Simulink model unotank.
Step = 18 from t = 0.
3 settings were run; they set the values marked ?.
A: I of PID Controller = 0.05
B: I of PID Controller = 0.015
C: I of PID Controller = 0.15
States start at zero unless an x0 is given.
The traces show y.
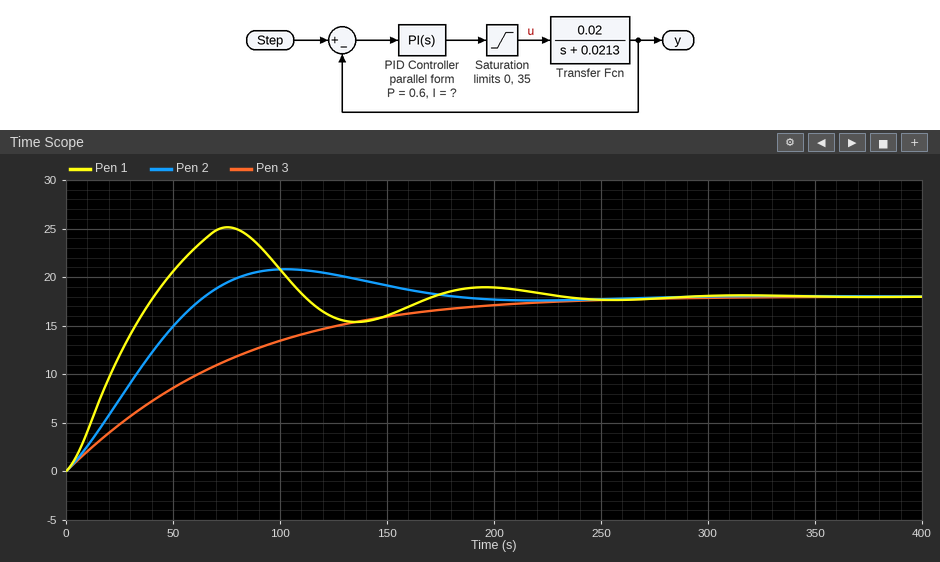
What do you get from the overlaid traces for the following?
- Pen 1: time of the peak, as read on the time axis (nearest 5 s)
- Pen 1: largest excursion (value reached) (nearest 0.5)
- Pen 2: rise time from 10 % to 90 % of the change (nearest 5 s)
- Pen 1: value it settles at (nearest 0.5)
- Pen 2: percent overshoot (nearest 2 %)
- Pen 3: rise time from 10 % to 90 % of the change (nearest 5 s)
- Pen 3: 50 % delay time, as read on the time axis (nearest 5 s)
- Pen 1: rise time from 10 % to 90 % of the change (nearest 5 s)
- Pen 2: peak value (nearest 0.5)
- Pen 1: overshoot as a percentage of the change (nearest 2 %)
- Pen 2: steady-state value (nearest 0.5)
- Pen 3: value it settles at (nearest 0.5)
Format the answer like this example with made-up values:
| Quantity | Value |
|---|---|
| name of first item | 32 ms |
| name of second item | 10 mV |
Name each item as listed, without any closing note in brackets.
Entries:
| Quantity | Value |
|---|---|
| Pen 1: time of the peak, as read on the time axis | 75 s |
| Pen 1: largest excursion (value reached) | 25.0 |
| Pen 2: rise time from 10 % to 90 % of the change | 50 s |
| Pen 1: value it settles at | 18.0 |
| Pen 2: percent overshoot | 16 % |
| Pen 3: rise time from 10 % to 90 % of the change | 150 s |
| Pen 3: 50 % delay time, as read on the time axis | 55 s |
| Pen 1: rise time from 10 % to 90 % of the change | 30 s |
| Pen 2: peak value | 21.0 |
| Pen 1: overshoot as a percentage of the change | 40 % |
| Pen 2: steady-state value | 18.0 |
| Pen 3: value it settles at | 18.0 |
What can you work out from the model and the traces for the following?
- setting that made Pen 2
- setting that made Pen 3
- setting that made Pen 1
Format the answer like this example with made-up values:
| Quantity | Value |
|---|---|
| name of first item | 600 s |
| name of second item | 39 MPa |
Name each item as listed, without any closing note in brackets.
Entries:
| Quantity | Value |
|---|---|
| setting that made Pen 2 | A |
| setting that made Pen 3 | B |
| setting that made Pen 1 | C |
